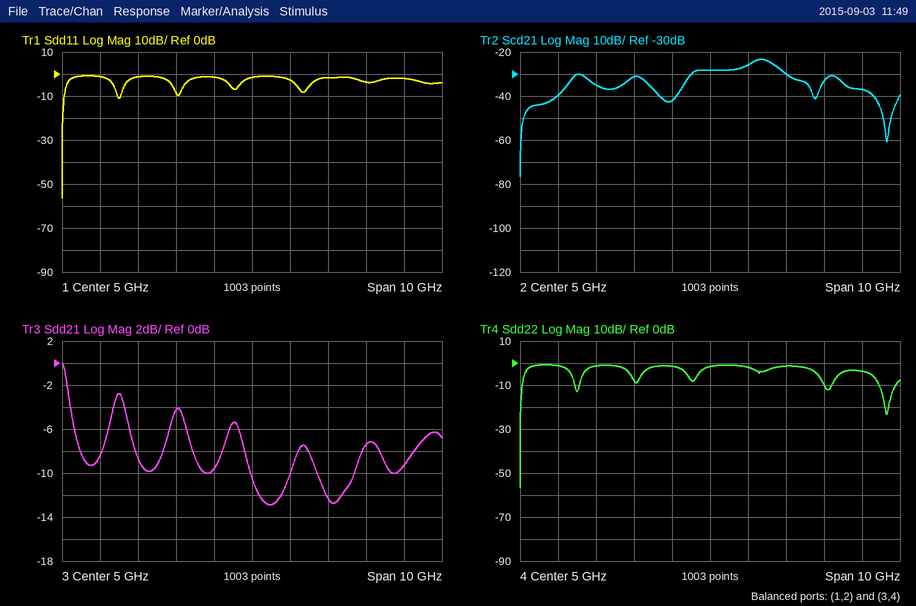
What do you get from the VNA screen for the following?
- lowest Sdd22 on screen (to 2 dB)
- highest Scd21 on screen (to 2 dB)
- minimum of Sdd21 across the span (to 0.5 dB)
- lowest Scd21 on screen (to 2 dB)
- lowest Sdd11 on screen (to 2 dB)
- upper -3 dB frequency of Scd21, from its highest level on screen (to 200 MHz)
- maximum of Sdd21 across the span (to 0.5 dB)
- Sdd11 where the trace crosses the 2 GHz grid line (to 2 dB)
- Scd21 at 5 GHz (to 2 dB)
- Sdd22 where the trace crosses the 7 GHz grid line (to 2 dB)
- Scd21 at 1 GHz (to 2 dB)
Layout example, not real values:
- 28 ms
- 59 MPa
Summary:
- -56 dB
- -24 dB
- -13.0 dB
- -76 dB
- -56 dB
- 6.8 GHz
- 0.0 dB
- -2 dB
- -28 dB
- -2 dB
- -40 dB
